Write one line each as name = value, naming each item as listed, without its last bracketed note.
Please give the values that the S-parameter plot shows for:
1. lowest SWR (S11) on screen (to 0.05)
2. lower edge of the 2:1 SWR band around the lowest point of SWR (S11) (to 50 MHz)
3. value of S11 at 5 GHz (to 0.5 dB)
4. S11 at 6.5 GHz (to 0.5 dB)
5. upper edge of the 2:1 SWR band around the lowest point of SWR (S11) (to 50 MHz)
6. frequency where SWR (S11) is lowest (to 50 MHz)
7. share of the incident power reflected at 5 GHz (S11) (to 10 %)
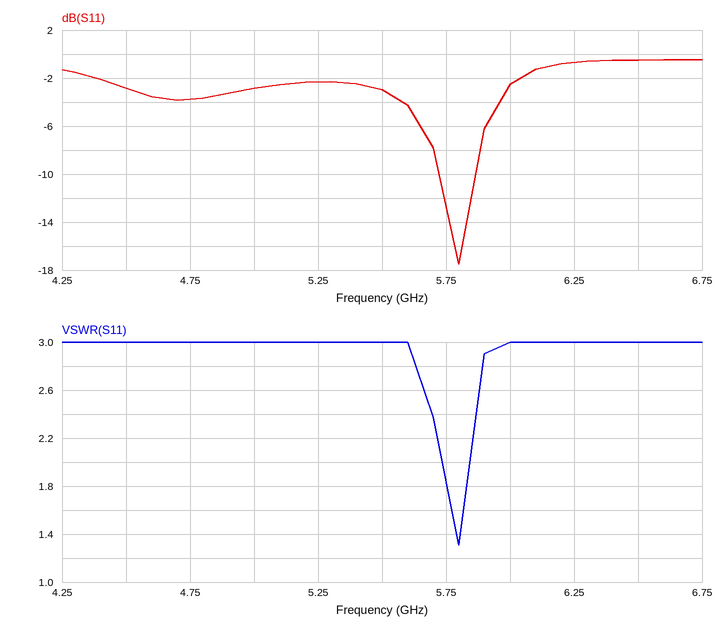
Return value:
lowest SWR (S11) on screen = 1.30
lower edge of the 2:1 SWR band around the lowest point of SWR (S11) = 5.75 GHz
value of S11 at 5 GHz = -3.0 dB
S11 at 6.5 GHz = -0.5 dB
upper edge of the 2:1 SWR band around the lowest point of SWR (S11) = 5.85 GHz
frequency where SWR (S11) is lowest = 5.80 GHz
share of the incident power reflected at 5 GHz (S11) = 50 %
